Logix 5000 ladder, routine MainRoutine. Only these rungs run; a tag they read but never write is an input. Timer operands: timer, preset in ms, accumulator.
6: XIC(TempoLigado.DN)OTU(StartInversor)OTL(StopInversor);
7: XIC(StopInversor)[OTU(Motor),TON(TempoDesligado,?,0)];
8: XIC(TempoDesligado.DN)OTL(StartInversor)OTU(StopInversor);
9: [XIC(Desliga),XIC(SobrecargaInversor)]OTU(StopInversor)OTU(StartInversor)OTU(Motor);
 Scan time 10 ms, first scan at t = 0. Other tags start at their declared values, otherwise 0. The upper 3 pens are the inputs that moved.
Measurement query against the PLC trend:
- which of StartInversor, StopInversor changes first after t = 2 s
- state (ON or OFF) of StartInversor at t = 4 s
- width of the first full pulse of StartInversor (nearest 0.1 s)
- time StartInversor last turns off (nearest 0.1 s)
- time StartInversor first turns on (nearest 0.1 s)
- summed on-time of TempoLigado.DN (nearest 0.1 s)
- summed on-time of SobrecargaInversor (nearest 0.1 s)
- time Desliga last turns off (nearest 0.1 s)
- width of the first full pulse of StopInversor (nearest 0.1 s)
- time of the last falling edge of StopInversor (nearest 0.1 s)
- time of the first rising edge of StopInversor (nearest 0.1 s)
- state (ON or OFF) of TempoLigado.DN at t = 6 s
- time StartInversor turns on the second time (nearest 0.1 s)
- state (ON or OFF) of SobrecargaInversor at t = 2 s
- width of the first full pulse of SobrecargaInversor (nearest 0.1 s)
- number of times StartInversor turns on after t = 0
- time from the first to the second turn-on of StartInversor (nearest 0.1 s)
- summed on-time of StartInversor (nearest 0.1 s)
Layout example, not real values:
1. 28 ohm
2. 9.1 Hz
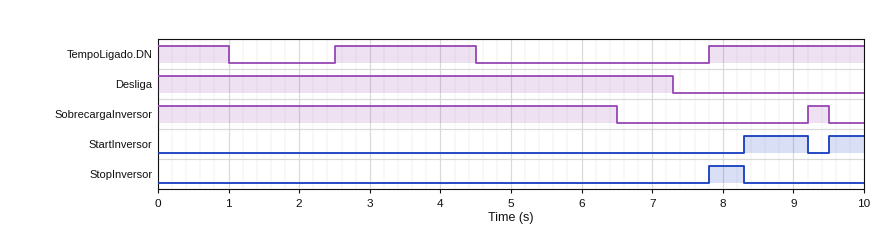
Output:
1. StopInversor
2. OFF
3. 0.9 s
4. 9.2 s
5. 8.3 s
6. 5.2 s
7. 6.8 s
8. 7.3 s
9. 0.5 s
10. 8.3 s
11. 7.8 s
12. OFF
13. 9.5 s
14. ON
15. 0.3 s
16. 2
17. 1.2 s
18. 1.4 s
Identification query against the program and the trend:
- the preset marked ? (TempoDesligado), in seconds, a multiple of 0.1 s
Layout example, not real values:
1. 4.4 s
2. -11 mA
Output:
1. 0.5 s
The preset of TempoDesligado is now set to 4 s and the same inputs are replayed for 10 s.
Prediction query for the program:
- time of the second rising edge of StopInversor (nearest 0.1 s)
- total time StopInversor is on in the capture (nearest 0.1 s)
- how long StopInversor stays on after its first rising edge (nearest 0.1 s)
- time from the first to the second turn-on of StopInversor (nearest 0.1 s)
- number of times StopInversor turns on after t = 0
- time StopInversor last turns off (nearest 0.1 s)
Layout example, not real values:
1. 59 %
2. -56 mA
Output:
1. 9.5 s
2. 1.9 s
3. 1.4 s
4. 1.7 s
5. 2
6. 9.2 s
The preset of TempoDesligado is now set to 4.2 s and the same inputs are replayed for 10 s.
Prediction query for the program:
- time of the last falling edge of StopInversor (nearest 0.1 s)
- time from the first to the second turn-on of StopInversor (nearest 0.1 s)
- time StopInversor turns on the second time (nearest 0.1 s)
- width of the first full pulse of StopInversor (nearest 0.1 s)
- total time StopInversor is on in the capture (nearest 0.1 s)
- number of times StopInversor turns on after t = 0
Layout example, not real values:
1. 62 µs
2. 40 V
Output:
1. 9.2 s
2. 1.7 s
3. 9.5 s
4. 1.4 s
5. 1.9 s
6. 2
